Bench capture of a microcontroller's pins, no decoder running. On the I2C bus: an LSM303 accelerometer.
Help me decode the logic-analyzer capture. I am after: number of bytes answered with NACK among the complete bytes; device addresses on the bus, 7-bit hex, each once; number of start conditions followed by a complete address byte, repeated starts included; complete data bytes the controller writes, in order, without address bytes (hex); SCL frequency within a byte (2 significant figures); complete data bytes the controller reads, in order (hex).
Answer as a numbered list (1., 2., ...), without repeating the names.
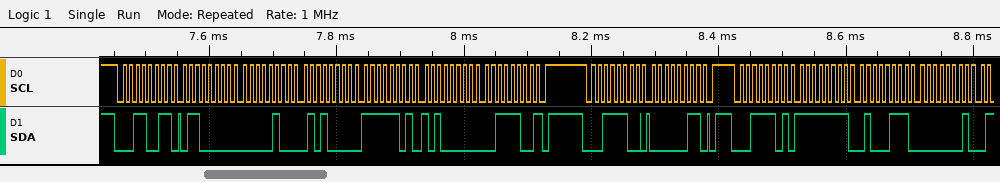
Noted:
1. 1
2. 0x19 0x1E
3. 3
4. 03
5. 100 kHz
6. 60 04 50 FD A0 3C FF 47 01
